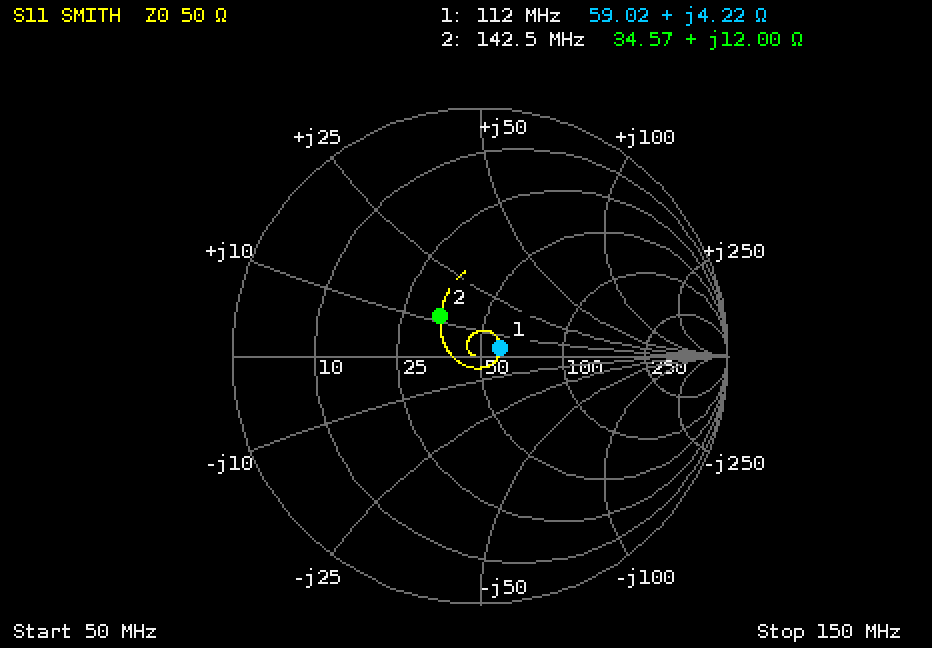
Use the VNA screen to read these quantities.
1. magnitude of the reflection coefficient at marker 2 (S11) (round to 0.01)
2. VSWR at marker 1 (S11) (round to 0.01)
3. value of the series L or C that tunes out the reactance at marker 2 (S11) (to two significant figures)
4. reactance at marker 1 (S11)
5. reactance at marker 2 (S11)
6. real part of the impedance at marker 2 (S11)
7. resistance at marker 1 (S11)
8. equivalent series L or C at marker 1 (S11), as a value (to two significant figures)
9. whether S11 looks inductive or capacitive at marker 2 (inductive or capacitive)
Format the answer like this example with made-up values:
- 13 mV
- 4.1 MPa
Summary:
- 0.23
- 1.20
- 93 pF
- +4.22 Ω
- +12.00 Ω
- 34.57 Ω
- 59.02 Ω
- 6.0 nH
- inductive
